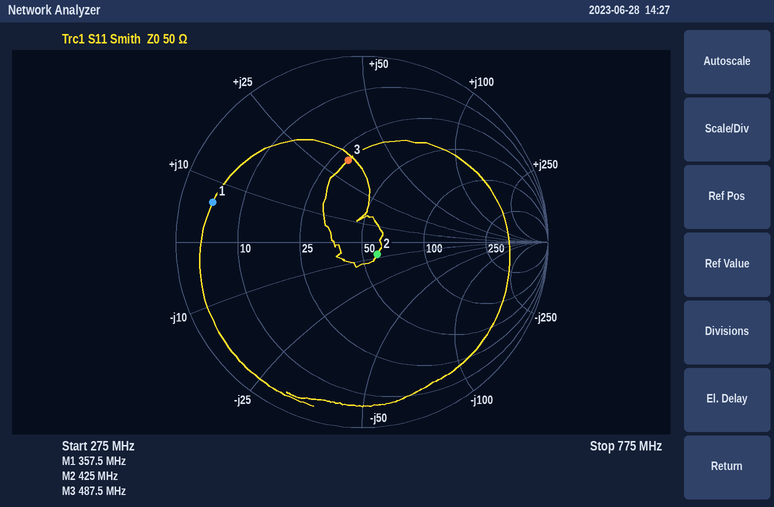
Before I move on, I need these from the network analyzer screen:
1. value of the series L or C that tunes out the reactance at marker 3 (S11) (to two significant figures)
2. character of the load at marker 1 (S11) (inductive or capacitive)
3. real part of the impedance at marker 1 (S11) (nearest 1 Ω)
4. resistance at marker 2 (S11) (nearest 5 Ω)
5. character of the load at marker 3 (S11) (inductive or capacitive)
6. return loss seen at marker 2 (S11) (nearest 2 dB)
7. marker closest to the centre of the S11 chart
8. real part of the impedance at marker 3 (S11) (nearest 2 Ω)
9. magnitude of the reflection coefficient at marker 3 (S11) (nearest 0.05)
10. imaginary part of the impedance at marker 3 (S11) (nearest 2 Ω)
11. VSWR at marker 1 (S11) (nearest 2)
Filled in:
10 pF
inductive
5 Ω
60 Ω
inductive
20 dB
marker 2
30 Ω
0.45
+32 Ω
10
